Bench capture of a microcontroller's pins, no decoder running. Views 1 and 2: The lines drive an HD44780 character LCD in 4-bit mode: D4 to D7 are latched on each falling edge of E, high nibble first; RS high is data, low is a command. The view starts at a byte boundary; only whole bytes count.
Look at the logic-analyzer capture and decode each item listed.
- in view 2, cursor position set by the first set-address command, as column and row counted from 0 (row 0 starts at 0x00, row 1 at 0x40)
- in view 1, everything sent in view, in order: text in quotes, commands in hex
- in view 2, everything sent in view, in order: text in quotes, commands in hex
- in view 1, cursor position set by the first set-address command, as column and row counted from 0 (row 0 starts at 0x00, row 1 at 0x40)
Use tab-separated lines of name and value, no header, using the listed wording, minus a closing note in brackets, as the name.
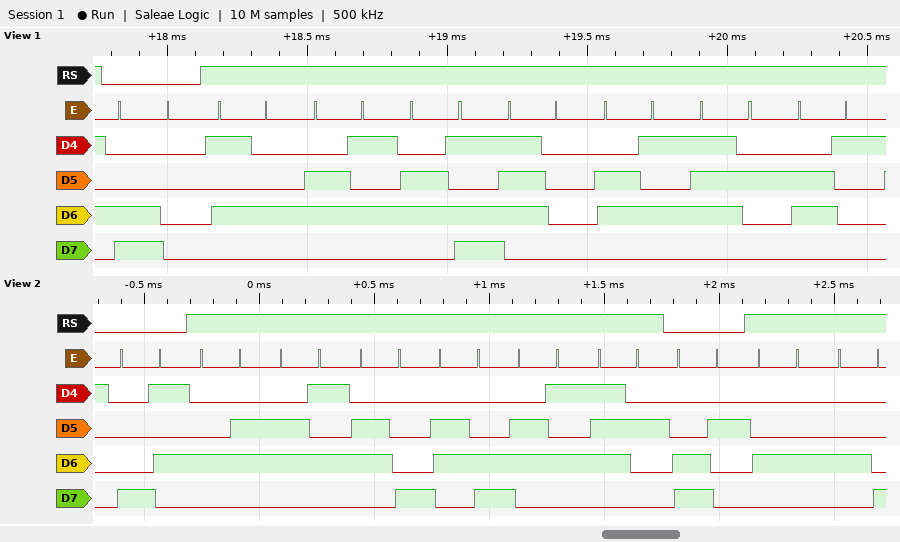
in view 2, cursor position set by the first set-address command, as column and row counted from 0	column 5, row 0
in view 1, everything sent in view, in order: text in quotes, commands in hex	0xC0 "Tempera"
in view 2, everything sent in view, in order: text in quotes, commands in hex	0x85 "Fehler" 0xC2 "DH"
in view 1, cursor position set by the first set-address command, as column and row counted from 0	column 0, row 1
